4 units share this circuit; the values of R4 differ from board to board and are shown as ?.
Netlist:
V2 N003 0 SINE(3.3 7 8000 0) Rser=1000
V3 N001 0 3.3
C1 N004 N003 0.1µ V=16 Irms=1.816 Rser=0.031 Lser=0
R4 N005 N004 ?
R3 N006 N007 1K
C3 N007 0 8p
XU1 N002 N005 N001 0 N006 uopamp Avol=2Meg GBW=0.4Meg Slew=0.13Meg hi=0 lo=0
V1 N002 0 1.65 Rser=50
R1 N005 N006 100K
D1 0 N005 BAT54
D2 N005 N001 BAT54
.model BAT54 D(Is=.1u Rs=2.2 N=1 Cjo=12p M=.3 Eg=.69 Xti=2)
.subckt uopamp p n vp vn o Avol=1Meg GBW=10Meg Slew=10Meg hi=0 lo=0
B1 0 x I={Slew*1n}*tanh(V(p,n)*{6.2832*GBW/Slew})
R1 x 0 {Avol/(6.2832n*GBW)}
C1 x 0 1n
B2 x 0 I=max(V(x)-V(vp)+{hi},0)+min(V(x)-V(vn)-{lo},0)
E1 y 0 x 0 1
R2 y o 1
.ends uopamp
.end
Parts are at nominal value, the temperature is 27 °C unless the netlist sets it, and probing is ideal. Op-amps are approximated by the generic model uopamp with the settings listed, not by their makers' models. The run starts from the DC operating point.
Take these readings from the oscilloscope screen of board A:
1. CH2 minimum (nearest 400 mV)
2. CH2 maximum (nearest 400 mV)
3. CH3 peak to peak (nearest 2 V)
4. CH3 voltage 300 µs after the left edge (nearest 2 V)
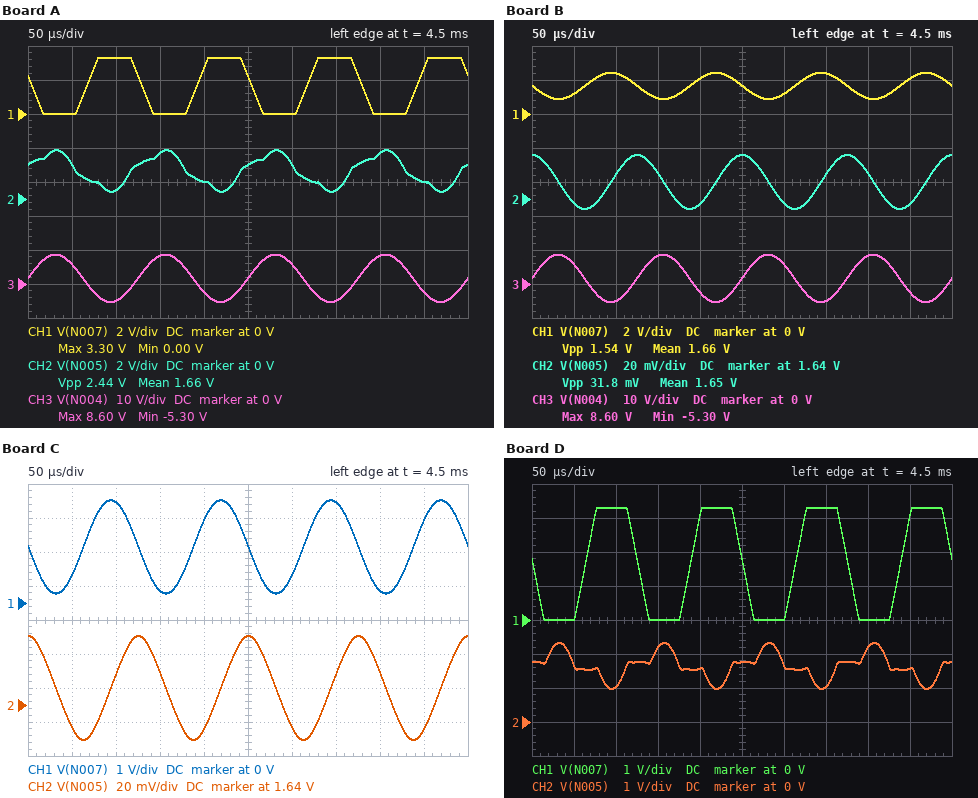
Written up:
400 mV
2.8 V
14 V
6 V
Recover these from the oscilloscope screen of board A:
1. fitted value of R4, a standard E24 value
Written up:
200 kΩ
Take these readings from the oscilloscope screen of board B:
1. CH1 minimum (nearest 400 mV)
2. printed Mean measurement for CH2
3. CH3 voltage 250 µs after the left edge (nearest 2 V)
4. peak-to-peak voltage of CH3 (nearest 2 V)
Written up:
800 mV
1.65 V
2 V
14 V
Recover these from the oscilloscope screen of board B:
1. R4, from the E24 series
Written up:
910 kΩ
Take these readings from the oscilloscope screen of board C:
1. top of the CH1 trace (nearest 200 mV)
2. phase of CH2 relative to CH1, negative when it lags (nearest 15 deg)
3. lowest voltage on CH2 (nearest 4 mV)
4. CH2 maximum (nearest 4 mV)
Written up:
3.0 V
-90 deg
1.620 V
1.680 V
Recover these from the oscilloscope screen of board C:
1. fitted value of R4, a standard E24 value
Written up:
510 kΩ
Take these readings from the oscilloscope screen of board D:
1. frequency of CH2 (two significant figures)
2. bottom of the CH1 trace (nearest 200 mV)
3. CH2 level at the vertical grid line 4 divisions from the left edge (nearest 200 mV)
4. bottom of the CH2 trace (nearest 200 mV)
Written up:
8.0 kHz
0 V
1.6 V
1.0 V
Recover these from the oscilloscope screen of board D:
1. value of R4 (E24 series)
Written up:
270 kΩ
